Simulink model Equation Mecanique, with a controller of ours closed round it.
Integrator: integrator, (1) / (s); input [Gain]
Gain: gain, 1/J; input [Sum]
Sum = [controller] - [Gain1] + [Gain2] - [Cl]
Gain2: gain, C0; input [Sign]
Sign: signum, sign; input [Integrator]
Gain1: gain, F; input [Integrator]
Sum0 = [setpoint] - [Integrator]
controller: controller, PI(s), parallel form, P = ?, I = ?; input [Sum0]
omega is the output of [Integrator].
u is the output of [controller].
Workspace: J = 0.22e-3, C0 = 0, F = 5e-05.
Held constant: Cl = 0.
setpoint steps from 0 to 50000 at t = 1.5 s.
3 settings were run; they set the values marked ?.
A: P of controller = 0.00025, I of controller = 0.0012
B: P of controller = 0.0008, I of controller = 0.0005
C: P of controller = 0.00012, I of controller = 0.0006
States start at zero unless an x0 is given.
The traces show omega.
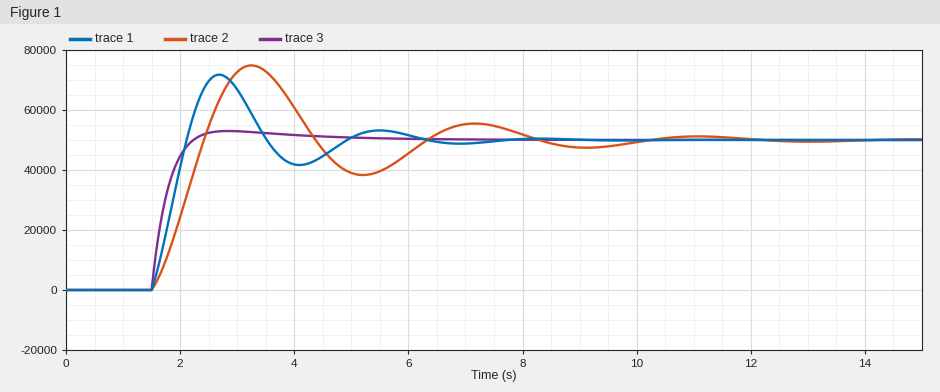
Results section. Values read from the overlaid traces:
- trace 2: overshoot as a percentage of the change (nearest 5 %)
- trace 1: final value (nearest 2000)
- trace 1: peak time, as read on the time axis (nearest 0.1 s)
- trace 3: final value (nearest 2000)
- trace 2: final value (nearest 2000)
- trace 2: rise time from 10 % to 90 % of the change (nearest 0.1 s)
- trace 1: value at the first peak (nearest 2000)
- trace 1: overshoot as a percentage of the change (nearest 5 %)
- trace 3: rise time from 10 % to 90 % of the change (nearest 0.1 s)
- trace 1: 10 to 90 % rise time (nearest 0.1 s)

50 %
50000
2.7 s
50000
50000
0.7 s
72000
45 %
0.5 s
0.5 s
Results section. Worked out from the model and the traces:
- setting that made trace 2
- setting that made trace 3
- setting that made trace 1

C
B
A
